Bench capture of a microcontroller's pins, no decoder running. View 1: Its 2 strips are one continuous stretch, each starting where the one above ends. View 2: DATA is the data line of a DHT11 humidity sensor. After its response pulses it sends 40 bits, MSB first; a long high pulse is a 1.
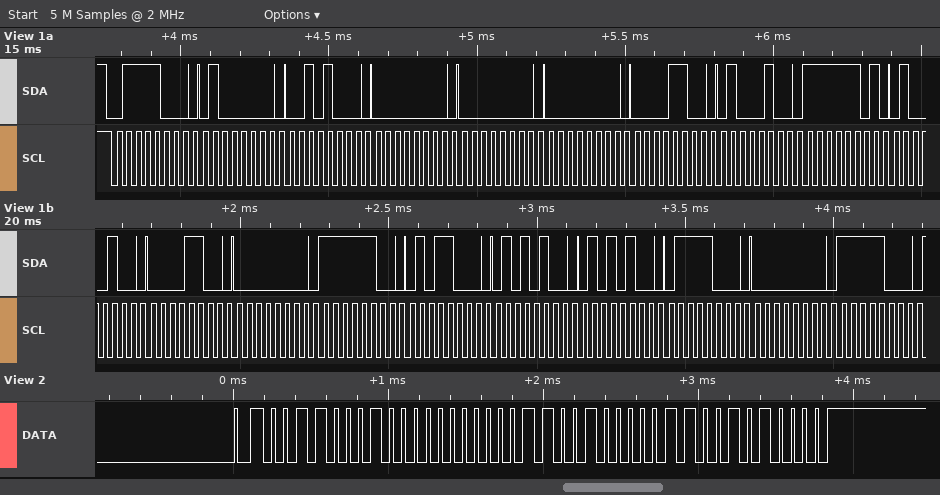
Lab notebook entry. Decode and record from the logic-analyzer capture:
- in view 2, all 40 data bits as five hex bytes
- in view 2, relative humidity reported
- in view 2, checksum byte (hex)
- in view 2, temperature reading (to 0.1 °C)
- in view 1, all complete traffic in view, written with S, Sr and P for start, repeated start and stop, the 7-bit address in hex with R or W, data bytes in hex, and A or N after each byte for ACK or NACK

31 00 19 06 50
49 %
0x50
25.6 °C
S 3CW A 40 A 28 A 00 A 00 A 00 A 0C A 44 A FD A 44 A 0C A 00 A FC A 58 A 54 A 54 A 78 A 00 A F8 A
